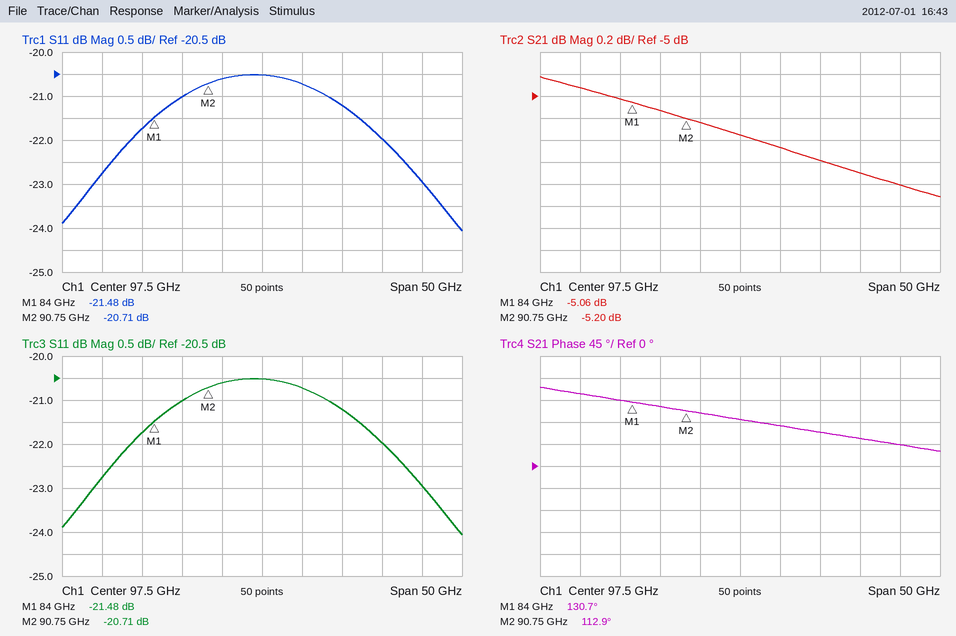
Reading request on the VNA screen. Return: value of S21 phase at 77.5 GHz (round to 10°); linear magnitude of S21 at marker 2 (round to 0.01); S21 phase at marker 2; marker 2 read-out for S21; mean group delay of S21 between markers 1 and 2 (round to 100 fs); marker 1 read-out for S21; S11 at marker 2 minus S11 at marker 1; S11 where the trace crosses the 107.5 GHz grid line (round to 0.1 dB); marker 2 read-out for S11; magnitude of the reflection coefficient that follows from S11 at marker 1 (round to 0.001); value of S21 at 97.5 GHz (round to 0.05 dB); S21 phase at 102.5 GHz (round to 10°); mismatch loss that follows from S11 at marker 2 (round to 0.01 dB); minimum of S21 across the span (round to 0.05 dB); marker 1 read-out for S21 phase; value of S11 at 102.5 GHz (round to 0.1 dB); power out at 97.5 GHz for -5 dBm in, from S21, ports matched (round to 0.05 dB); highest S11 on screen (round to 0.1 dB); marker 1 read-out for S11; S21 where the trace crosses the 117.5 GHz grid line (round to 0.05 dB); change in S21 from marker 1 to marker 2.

150°
0.55
112.9°
-5.20 dB
7.3 ps
-5.06 dB
0.77 dB
-21.2 dB
-20.71 dB
0.084
-5.35 dB
80°
0.04 dB
-5.90 dB
130.7°
-20.7 dB
-10.35 dBm
-20.5 dB
-21.48 dB
-5.80 dB
-0.14 dB
